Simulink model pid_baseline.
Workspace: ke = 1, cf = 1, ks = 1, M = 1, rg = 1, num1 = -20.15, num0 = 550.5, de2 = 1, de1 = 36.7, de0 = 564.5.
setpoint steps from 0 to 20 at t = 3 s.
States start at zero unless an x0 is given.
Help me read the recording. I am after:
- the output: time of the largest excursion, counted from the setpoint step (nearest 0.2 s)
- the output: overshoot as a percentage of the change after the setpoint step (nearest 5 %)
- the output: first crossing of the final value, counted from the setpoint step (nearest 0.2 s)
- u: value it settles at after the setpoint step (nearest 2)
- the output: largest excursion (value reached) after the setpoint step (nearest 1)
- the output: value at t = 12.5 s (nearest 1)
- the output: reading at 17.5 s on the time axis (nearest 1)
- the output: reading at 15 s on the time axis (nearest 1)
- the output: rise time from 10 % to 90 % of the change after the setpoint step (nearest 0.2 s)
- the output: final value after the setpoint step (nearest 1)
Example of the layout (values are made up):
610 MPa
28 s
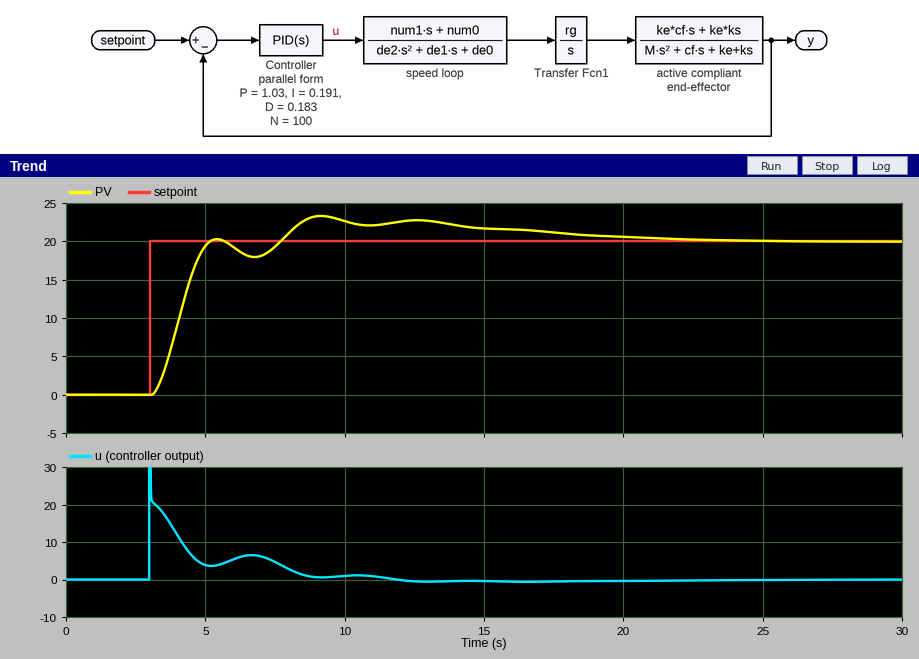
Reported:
6.2 s
15 %
2.2 s
0
23
23
21
22
1.4 s
20
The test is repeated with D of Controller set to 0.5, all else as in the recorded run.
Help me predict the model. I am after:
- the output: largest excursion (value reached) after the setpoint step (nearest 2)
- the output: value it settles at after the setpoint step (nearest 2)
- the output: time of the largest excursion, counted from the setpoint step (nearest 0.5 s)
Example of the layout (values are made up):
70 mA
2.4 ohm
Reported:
22
20
9.0 s
